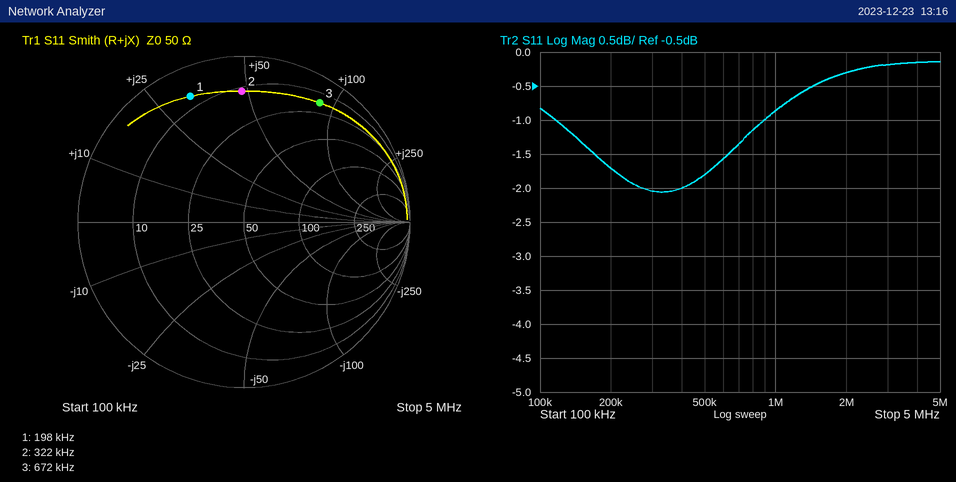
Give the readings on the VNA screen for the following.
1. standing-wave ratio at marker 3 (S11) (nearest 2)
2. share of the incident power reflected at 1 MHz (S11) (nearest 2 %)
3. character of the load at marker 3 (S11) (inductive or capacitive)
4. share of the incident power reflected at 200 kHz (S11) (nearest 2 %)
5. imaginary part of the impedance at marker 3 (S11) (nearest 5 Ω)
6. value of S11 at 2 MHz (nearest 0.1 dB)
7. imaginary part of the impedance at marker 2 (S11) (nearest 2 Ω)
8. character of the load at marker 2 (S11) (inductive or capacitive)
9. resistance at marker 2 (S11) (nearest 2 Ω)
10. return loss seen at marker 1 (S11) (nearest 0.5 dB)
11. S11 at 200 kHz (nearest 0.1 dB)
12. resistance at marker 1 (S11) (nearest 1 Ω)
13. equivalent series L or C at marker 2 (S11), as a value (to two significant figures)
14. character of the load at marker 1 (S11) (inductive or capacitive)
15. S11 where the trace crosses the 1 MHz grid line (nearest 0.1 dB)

12
82 %
inductive
68 %
+90 Ω
-0.3 dB
+48 Ω
inductive
12 Ω
1.5 dB
-1.7 dB
7 Ω
24 µH
inductive
-0.9 dB
